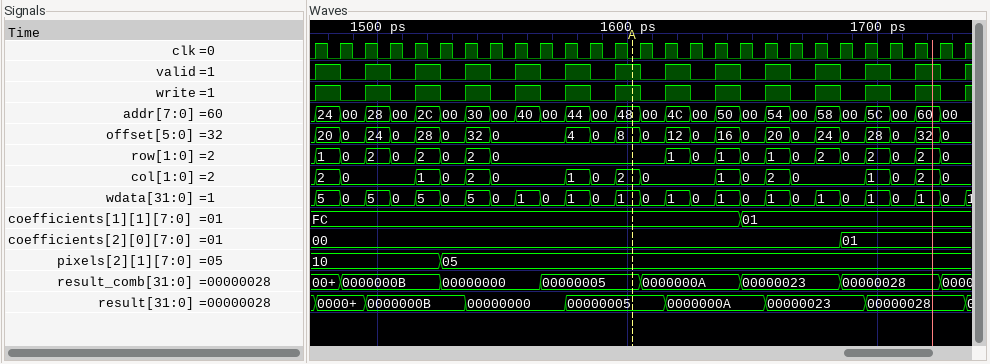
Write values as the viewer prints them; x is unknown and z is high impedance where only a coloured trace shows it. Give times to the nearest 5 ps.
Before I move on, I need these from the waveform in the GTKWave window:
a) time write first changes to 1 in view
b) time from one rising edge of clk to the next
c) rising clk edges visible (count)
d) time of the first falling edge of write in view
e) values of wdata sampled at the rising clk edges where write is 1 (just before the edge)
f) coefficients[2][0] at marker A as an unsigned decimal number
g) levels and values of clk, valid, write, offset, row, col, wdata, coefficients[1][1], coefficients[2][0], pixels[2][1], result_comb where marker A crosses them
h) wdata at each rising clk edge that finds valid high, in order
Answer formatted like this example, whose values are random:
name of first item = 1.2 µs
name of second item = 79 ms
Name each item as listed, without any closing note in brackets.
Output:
time write first changes to 1 in view = 1475 ps
time from one rising edge of clk to the next = 10 ps
rising clk edges visible = 27
time of the first falling edge of write in view = 1485 ps
values of wdata sampled at the rising clk edges where write is 1 = 5, 5, 5, 5, 1, 1, 1, 1, 1, 1, 1, 1, 1
coefficients[2][0] at marker A as an unsigned decimal number = 0
levels and values of clk, valid, write, offset, row, col, wdata, coefficients[1][1], coefficients[2][0], pixels[2][1], result_comb where marker A crosses them = clk=0, valid=1, write=1, offset=8, row=0, col=2, wdata=1, coefficients[1][1]=FC, coefficients[2][0]=00, pixels[2][1]=05, result_comb=00000005
wdata at each rising clk edge that finds valid high, in order = 5, 5, 5, 5, 1, 1, 1, 1, 1, 1, 1, 1, 1
